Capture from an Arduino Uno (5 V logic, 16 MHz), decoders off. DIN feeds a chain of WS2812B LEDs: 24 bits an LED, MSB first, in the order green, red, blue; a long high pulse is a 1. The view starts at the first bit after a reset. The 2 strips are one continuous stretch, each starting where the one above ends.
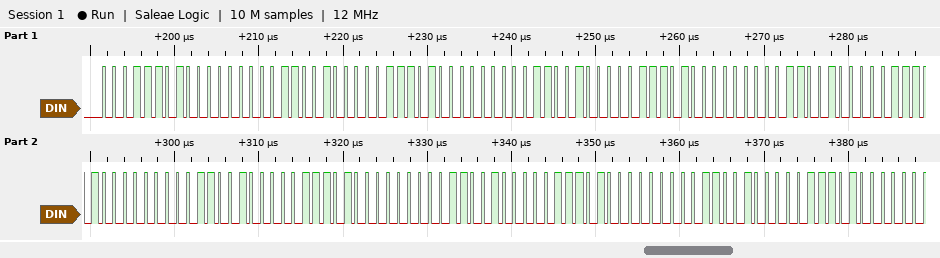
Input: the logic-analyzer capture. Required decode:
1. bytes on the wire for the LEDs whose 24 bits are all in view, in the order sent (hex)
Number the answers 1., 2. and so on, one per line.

1. 1D 00 64 1D 00 64 1D 00 64 1D 00 64 1D 00 64 1D 00 64
